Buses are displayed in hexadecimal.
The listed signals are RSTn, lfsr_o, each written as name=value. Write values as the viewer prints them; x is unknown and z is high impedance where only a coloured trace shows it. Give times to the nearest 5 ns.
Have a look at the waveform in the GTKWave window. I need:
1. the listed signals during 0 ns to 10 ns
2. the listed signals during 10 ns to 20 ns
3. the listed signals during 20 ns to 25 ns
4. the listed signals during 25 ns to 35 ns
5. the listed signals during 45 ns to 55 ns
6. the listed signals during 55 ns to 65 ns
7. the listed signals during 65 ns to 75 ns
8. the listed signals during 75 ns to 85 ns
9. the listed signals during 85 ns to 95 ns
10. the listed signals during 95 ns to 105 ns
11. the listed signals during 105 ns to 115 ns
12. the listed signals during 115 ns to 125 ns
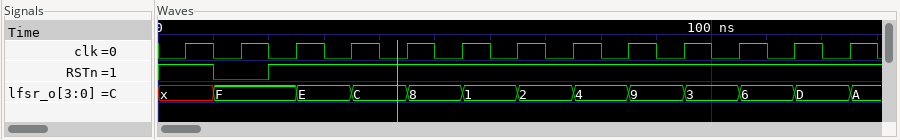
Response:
RSTn=1, lfsr_o=x
RSTn=0, lfsr_o=F
RSTn=1, lfsr_o=F
RSTn=1, lfsr_o=E
RSTn=1, lfsr_o=8
RSTn=1, lfsr_o=1
RSTn=1, lfsr_o=2
RSTn=1, lfsr_o=4
RSTn=1, lfsr_o=9
RSTn=1, lfsr_o=3
RSTn=1, lfsr_o=6
RSTn=1, lfsr_o=D
